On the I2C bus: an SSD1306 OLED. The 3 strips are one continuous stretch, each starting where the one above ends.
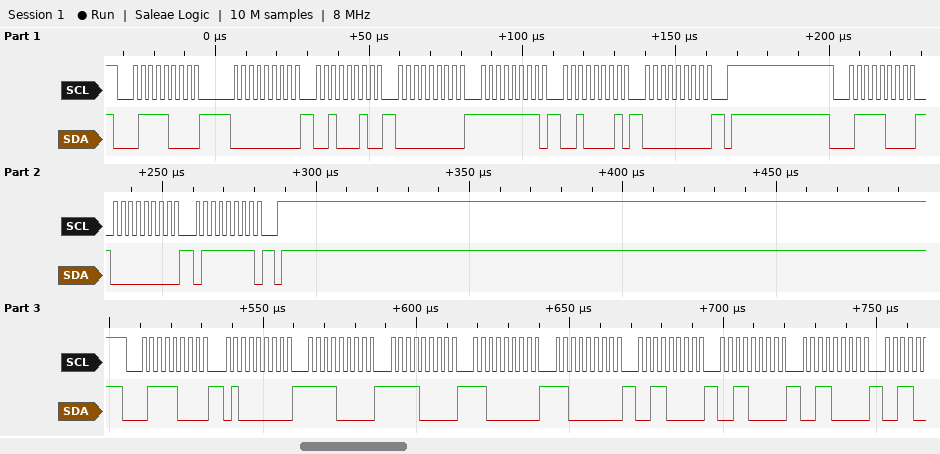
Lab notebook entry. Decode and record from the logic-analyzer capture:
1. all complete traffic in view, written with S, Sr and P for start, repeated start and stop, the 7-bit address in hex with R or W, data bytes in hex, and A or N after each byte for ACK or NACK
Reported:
S 3CW A 00 A 22 A 00 A FF A 21 A 00 A P S 3CW A 00 A 7F A P S 3CW A 40 A F0 A F0 A C0 A C0 A 30 A 30 A 30 A
